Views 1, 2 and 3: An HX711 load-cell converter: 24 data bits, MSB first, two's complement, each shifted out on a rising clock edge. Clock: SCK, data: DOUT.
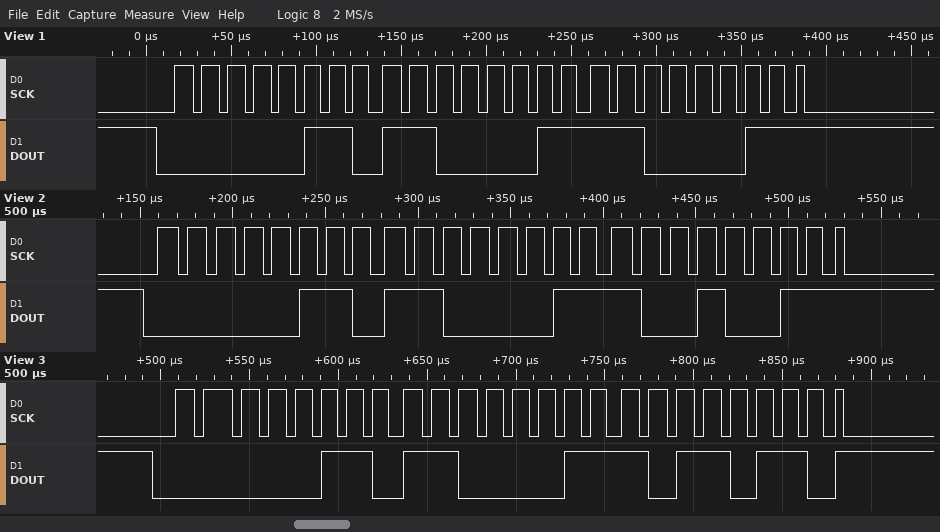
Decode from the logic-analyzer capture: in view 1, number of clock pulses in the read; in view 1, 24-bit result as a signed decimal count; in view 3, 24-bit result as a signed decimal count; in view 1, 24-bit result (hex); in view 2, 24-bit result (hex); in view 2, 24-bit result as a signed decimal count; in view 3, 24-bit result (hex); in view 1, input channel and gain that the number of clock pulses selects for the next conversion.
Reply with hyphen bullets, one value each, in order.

- 25
- 443331
- 443318
- 0x06C3C3
- 0x06C393
- 443283
- 0x06C3B6
- channel A, gain 128
